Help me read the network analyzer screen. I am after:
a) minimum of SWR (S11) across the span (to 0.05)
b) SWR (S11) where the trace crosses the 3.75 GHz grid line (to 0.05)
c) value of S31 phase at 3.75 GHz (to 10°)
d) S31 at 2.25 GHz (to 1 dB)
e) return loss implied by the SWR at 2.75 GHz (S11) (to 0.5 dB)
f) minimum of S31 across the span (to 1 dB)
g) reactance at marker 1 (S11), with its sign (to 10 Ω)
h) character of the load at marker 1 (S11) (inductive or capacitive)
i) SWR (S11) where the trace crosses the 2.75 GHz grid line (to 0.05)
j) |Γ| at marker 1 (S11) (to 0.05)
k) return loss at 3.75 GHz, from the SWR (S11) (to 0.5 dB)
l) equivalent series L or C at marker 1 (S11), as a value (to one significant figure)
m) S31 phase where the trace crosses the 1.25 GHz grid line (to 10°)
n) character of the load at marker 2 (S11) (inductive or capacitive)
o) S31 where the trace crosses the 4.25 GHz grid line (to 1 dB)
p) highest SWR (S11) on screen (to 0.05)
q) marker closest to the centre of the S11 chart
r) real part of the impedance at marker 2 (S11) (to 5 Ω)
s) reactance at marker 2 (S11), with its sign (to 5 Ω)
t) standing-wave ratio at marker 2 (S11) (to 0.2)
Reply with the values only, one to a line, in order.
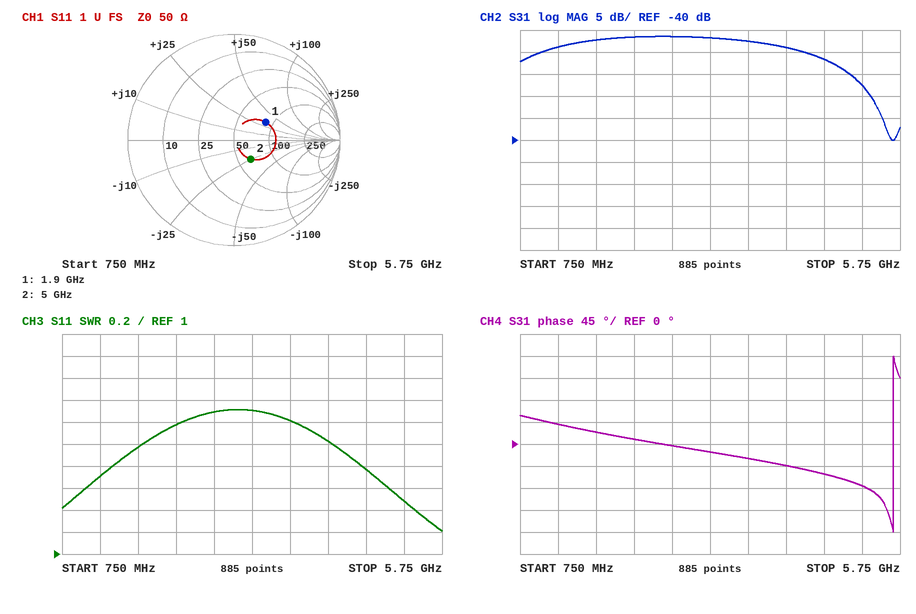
1.20
2.20
-30°
-17 dB
8.0 dB
-40 dB
+30 Ω
inductive
2.30
0.35
8.5 dB
3 nH
40°
capacitive
-19 dB
2.30
marker 2
65 Ω
-25 Ω
1.6
